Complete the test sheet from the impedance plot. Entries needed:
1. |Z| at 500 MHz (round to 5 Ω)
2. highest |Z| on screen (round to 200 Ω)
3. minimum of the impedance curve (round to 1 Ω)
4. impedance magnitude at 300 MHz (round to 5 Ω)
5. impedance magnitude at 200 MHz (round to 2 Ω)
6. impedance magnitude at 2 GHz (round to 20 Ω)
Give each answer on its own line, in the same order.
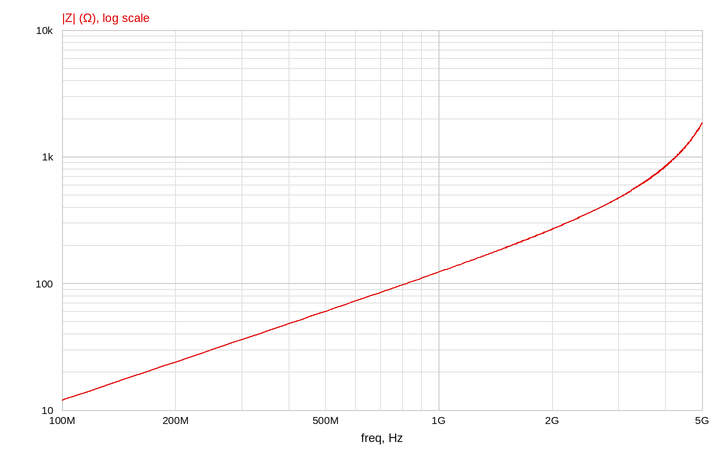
60 Ω
1.8 kΩ
12 Ω
35 Ω
24 Ω
260 Ω
